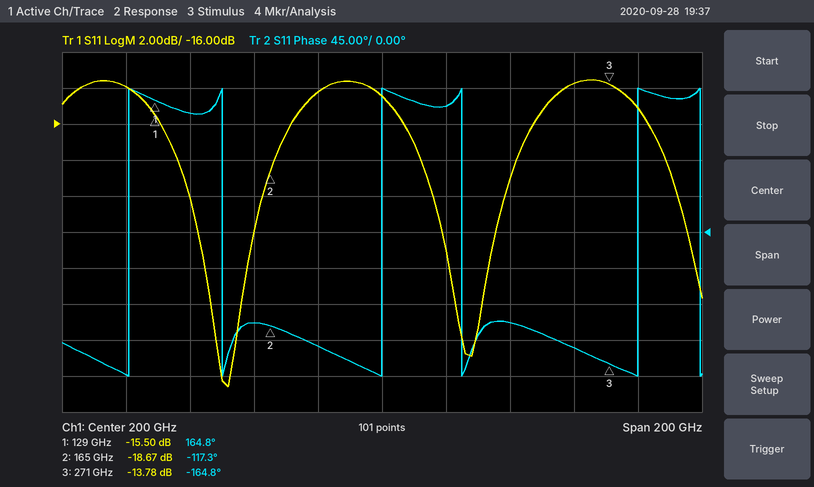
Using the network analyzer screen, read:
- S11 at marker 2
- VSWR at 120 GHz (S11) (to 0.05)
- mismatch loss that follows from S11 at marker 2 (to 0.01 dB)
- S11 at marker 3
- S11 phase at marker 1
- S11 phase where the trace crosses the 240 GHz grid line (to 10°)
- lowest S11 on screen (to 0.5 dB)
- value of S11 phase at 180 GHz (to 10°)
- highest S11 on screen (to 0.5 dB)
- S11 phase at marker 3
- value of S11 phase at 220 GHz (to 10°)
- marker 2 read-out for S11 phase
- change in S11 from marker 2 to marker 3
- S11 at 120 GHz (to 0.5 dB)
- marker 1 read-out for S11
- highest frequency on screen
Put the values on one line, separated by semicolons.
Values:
-18.67 dB; 1.50; 0.06 dB; -13.78 dB; 164.8°; -110°; -30.5 dB; -140°; -13.5 dB; -164.8°; 160°; -117.3°; 4.89 dB; -14.0 dB; -15.50 dB; 300 GHz
